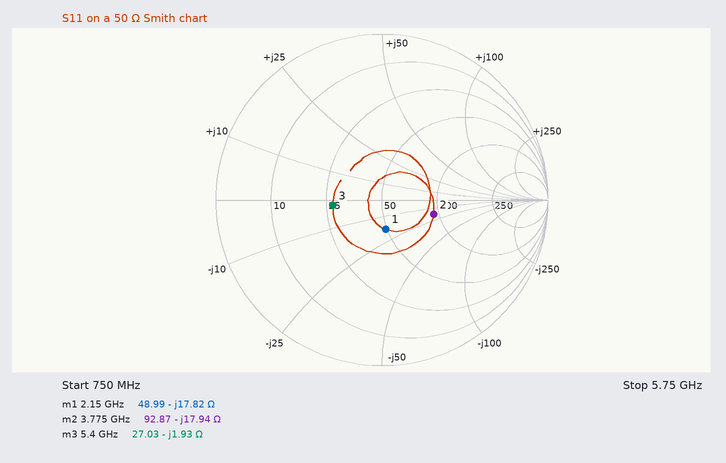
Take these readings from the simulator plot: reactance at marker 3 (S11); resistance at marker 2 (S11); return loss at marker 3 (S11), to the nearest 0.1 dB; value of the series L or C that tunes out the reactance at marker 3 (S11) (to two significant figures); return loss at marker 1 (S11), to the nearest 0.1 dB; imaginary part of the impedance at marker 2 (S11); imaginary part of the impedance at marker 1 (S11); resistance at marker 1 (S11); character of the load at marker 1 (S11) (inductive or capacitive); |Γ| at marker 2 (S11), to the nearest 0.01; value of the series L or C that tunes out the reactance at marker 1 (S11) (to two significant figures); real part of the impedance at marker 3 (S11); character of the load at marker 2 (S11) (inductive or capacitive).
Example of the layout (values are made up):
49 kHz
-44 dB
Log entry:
-1.93 Ω
92.87 Ω
10.5 dB
57 pH
15.0 dB
-17.94 Ω
-17.82 Ω
48.99 Ω
capacitive
0.32
1.3 nH
27.03 Ω
capacitive
